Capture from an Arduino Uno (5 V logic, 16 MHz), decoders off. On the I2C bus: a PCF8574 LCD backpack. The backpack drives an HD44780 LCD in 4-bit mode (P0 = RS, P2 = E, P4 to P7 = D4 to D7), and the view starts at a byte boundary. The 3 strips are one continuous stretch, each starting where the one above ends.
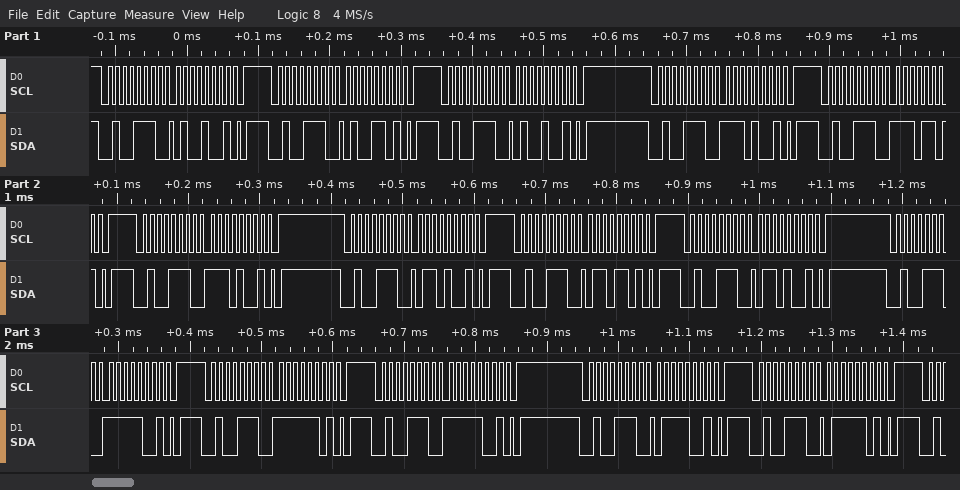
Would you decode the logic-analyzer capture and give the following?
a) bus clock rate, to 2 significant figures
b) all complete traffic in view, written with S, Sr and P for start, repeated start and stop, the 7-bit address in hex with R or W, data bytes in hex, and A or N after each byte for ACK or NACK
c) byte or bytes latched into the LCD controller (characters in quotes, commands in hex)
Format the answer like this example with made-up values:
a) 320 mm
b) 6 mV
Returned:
a) 100 kHz
b) S 27W A 49 A P S 27W A 4D A P S 27W A 49 A P S 27W A E9 A P S 27W A ED A P S 27W A E9 A P S 27W A 69 A P S 27W A 6D A P S 27W A 69 A P S 27W A F9 A P S 27W A FD A P S 27W A F9 A P S 27W A 79 A P S 27W A 7D A P
c) 'N' 'o'
